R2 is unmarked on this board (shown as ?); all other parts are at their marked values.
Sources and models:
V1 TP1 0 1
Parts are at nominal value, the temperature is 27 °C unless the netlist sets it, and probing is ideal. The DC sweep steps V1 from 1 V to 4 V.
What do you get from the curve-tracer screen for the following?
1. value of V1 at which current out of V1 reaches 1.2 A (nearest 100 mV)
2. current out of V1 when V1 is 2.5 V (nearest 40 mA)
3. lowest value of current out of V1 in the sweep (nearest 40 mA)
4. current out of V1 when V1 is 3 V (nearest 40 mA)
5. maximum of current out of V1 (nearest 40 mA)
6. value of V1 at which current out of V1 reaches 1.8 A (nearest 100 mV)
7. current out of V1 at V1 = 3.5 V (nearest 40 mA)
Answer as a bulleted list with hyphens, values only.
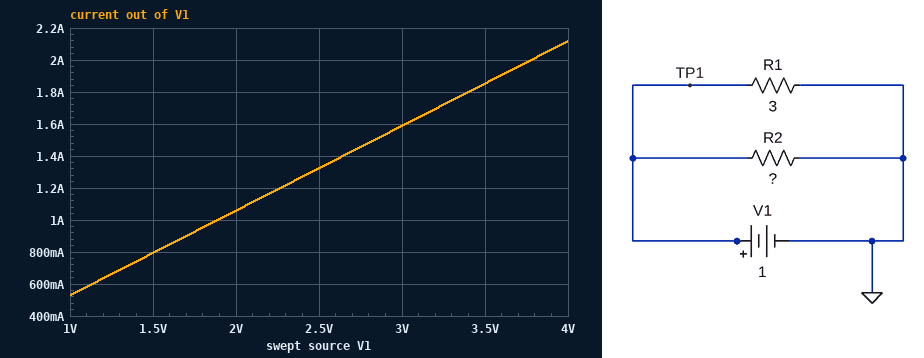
- 2.3 V
- 1.32 A
- 520 mA
- 1.60 A
- 2.12 A
- 3.4 V
- 1.84 A
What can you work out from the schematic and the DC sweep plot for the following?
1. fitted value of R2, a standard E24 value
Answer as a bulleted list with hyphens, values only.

- 5.1 Ω
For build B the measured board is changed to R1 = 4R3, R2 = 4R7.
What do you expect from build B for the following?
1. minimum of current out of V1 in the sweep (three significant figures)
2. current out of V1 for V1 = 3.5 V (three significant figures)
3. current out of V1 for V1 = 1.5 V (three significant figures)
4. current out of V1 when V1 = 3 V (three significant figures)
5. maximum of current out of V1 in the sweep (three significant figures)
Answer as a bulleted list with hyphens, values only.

- 445 mA
- 1.56 A
- 668 mA
- 1.34 A
- 1.78 A
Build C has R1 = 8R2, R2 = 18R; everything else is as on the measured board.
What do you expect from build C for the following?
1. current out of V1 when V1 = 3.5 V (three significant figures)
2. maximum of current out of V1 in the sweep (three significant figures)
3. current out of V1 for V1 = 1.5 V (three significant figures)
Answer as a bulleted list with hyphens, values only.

- 621 mA
- 710 mA
- 266 mA
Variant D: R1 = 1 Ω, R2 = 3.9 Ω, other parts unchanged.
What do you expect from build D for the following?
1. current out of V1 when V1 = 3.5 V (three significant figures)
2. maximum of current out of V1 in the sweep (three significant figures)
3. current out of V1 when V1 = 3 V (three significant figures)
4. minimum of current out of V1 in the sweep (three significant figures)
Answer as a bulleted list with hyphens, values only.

- 4.40 A
- 5.03 A
- 3.77 A
- 1.26 A
